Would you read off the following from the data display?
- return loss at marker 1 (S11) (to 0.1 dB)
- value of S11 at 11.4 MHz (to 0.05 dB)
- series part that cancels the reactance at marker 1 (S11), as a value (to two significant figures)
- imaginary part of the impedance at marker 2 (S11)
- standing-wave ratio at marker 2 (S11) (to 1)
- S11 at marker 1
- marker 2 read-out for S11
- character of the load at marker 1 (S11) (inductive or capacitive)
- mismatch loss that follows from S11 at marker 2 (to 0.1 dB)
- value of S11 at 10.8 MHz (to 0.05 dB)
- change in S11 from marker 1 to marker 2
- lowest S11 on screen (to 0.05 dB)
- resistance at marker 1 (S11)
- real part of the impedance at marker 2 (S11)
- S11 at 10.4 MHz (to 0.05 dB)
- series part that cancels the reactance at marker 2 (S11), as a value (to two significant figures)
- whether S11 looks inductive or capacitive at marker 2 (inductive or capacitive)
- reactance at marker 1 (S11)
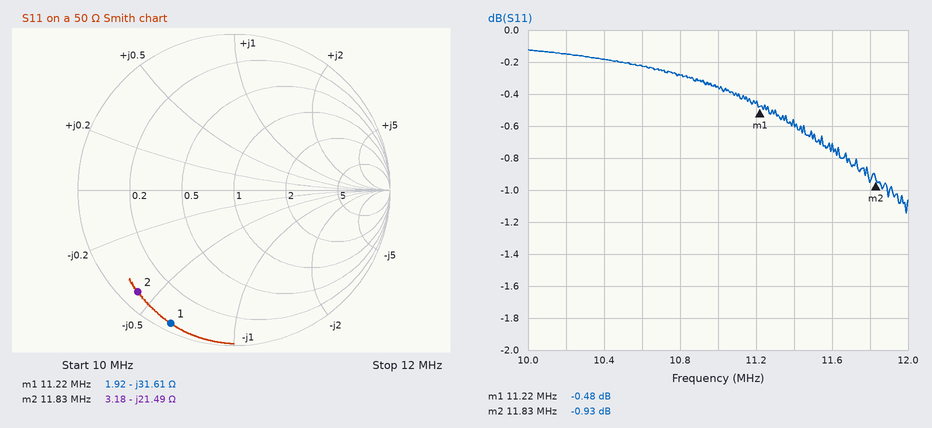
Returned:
0.5 dB
-0.60 dB
450 nH
-21.49 Ω
19
-0.48 dB
-0.93 dB
capacitive
7.1 dB
-0.30 dB
-0.45 dB
-1.15 dB
1.92 Ω
3.18 Ω
-0.20 dB
290 nH
capacitive
-31.61 Ω
